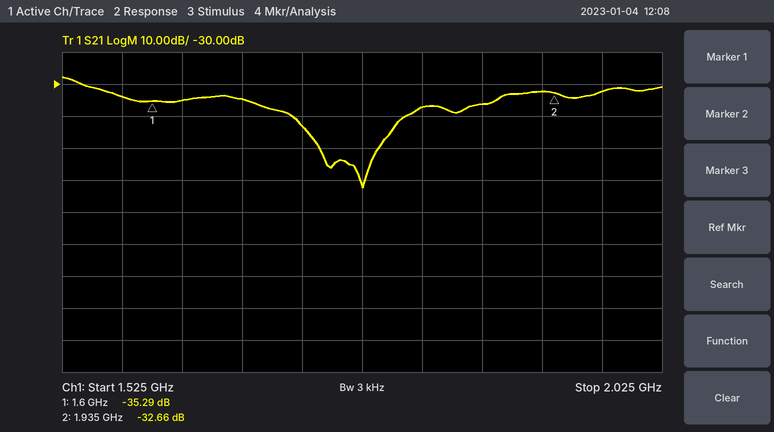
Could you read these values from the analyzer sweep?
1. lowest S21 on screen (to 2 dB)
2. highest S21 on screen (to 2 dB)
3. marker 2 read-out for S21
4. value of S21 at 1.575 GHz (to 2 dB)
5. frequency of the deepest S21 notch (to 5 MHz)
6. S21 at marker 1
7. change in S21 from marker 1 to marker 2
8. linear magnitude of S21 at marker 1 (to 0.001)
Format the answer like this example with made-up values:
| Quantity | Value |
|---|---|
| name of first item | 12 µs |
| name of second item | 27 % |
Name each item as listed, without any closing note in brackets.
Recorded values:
| Quantity | Value |
|---|---|
| lowest S21 on screen | -62 dB |
| highest S21 on screen | -28 dB |
| marker 2 read-out for S21 | -32.66 dB |
| value of S21 at 1.575 GHz | -34 dB |
| frequency of the deepest S21 notch | 1.775 GHz |
| S21 at marker 1 | -35.29 dB |
| change in S21 from marker 1 to marker 2 | 2.63 dB |
| linear magnitude of S21 at marker 1 | 0.017 |
